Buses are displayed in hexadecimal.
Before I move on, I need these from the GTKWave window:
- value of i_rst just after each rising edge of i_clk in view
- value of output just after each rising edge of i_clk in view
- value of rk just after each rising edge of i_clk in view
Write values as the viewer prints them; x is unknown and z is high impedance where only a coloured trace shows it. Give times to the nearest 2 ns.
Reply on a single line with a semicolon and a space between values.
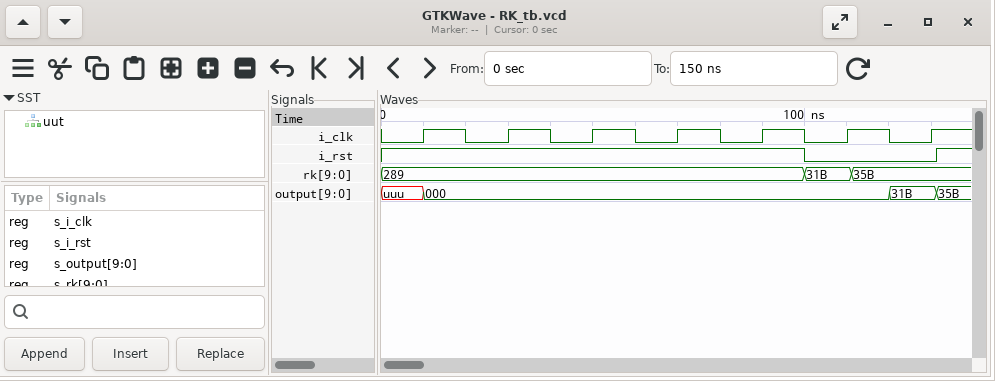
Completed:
1 1 1 1 1 0 0; 000, 000, 000, 000, 000, 000, 31B; 289, 289, 289, 289, 289, 31B, 35B
